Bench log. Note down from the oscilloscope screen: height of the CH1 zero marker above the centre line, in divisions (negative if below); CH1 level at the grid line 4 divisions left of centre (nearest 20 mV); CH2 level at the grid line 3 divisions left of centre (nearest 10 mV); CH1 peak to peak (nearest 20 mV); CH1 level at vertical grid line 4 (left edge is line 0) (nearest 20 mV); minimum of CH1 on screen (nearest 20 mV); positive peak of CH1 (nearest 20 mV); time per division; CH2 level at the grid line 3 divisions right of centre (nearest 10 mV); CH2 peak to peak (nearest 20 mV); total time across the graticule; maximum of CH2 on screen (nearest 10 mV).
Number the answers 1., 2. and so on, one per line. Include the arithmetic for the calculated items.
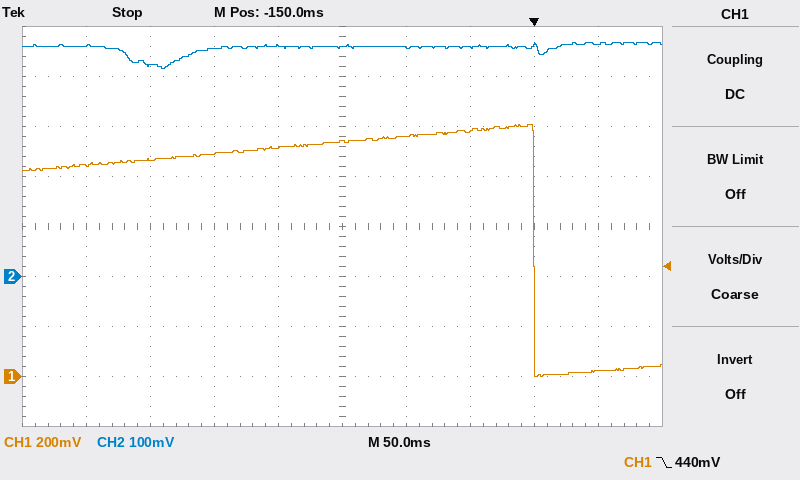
1. -3.0 div
2. 840 mV
3. 420 mV
4. 1.00 V − (0 mV) = 1.00 V
5. 920 mV
6. 0 mV
7. 1.00 V
8. 50 ms
9. 460 mV
10. 60 mV
11. 500 ms
12. 470 mV
